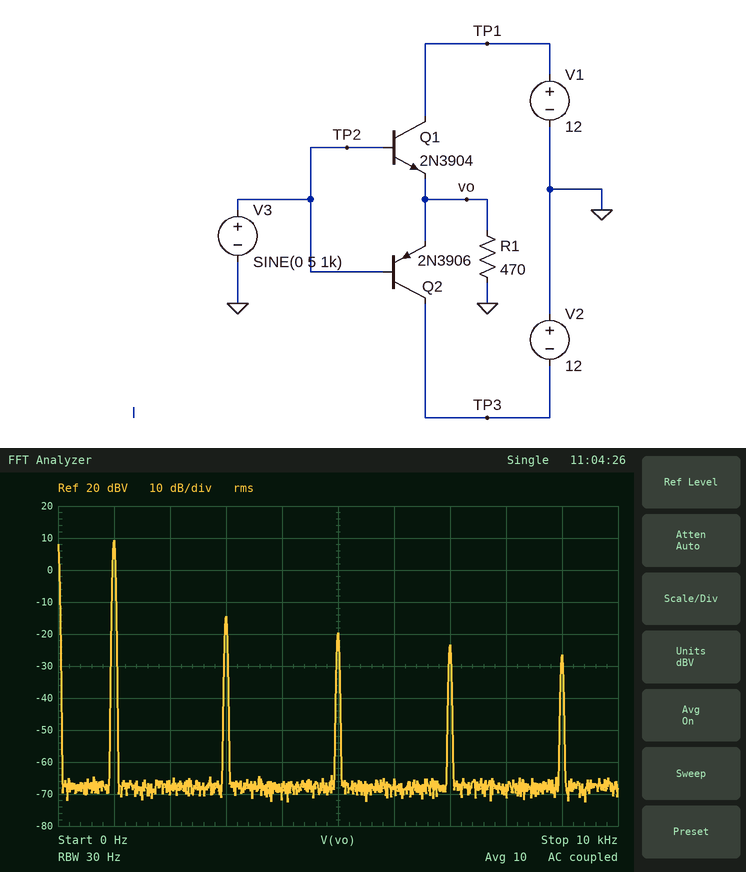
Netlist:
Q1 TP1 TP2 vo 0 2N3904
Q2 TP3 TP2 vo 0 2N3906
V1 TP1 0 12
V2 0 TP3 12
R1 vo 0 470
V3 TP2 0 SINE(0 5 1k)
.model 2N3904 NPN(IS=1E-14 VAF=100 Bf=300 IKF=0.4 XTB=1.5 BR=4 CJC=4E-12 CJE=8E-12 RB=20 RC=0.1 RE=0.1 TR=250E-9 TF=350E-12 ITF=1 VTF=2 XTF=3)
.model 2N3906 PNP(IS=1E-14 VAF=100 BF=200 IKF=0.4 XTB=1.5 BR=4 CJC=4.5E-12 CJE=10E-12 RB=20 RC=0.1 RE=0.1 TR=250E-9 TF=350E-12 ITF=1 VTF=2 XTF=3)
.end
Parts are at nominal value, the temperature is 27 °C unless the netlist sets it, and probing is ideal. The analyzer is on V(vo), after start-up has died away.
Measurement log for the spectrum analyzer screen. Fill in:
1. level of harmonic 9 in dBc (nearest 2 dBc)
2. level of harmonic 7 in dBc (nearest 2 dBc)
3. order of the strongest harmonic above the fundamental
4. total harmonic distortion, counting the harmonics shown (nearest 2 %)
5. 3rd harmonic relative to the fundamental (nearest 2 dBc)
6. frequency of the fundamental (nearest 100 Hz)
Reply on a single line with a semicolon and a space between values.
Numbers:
-36 dBc; -32 dBc; 3; 8 %; -24 dBc; 1.0 kHz
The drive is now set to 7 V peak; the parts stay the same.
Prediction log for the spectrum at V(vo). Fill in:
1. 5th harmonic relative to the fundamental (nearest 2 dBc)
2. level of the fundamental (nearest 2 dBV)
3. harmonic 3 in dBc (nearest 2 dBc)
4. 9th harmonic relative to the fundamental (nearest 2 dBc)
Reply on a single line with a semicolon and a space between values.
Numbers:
-32 dBc; 12 dBV; -26 dBc; -38 dBc
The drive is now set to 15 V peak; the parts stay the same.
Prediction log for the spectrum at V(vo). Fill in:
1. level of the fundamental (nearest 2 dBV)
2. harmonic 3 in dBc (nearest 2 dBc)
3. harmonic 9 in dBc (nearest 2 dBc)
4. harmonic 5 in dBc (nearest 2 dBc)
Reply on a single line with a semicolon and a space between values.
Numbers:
20 dBV; -28 dBc; -52 dBc; -26 dBc
